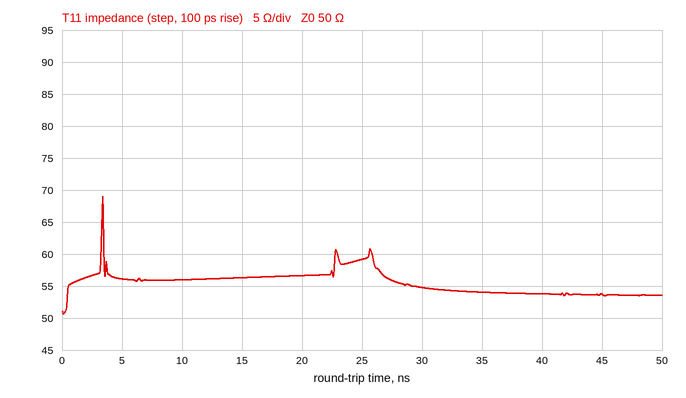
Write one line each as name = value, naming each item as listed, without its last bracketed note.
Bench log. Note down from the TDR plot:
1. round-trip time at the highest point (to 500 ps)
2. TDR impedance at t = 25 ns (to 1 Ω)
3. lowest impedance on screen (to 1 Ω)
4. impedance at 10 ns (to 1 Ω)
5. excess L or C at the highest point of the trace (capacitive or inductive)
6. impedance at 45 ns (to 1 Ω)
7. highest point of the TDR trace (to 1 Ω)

round-trip time at the highest point = 3.5 ns
TDR impedance at t = 25 ns = 59 Ω
lowest impedance on screen = 51 Ω
impedance at 10 ns = 56 Ω
excess L or C at the highest point of the trace = inductive
impedance at 45 ns = 54 Ω
highest point of the TDR trace = 69 Ω
